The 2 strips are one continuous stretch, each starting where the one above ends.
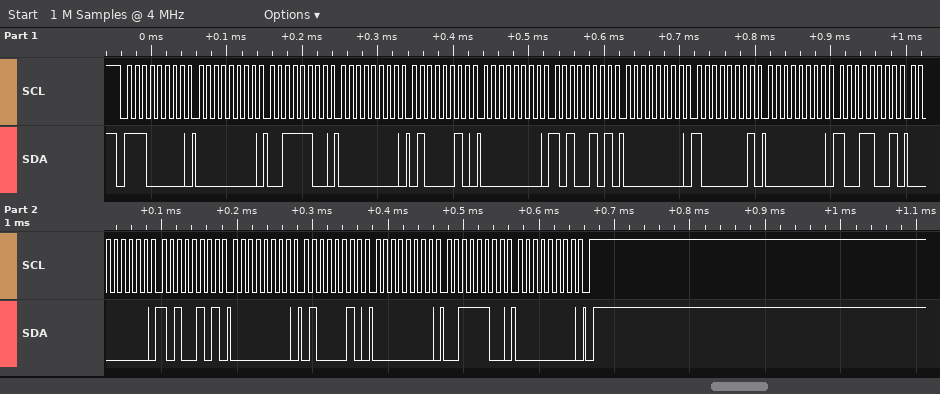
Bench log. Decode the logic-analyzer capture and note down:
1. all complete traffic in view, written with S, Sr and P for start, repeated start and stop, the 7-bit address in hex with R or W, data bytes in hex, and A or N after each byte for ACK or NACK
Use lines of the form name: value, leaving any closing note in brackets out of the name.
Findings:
all complete traffic in view, written with S, Sr and P for start, repeated start and stop, the 7-bit address in hex with R or W, data bytes in hex, and A or N after each byte for ACK or NACK: S 70W A 00 A 3C A 00 A 42 A 00 A A5 A 00 A 81 A 00 A 99 A 00 A A5 A 00 A 42 A 00 A 3C A 00 A P
